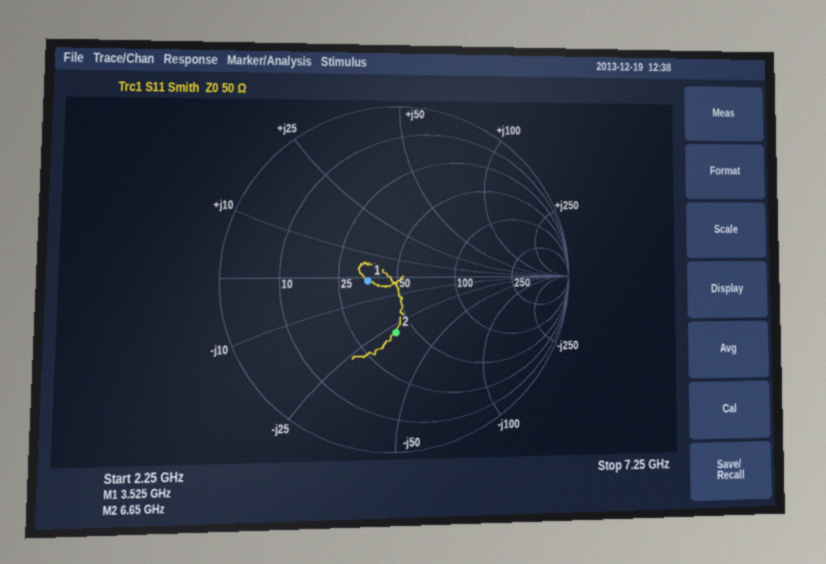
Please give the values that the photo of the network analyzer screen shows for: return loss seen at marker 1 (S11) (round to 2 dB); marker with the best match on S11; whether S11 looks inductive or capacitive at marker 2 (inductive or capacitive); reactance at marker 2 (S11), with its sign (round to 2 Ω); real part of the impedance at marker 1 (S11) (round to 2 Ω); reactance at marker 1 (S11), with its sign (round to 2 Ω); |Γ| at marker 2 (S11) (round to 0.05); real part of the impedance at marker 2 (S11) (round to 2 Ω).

16 dB
marker 1
capacitive
-28 Ω
36 Ω
-2 Ω
0.30
40 Ω
